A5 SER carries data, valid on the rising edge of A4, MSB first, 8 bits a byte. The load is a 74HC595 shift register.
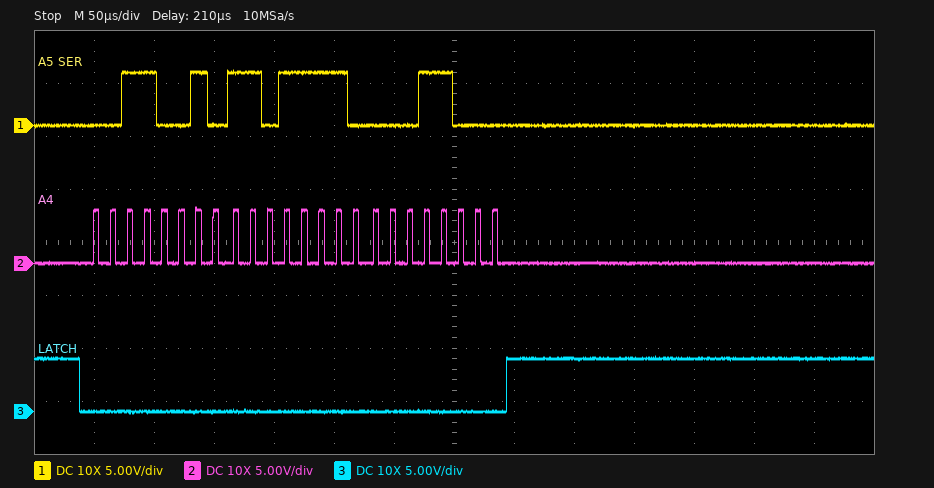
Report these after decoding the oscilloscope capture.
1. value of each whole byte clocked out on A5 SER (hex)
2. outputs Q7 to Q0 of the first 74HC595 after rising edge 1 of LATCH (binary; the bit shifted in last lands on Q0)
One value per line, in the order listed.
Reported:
32 DE 18
00011000
